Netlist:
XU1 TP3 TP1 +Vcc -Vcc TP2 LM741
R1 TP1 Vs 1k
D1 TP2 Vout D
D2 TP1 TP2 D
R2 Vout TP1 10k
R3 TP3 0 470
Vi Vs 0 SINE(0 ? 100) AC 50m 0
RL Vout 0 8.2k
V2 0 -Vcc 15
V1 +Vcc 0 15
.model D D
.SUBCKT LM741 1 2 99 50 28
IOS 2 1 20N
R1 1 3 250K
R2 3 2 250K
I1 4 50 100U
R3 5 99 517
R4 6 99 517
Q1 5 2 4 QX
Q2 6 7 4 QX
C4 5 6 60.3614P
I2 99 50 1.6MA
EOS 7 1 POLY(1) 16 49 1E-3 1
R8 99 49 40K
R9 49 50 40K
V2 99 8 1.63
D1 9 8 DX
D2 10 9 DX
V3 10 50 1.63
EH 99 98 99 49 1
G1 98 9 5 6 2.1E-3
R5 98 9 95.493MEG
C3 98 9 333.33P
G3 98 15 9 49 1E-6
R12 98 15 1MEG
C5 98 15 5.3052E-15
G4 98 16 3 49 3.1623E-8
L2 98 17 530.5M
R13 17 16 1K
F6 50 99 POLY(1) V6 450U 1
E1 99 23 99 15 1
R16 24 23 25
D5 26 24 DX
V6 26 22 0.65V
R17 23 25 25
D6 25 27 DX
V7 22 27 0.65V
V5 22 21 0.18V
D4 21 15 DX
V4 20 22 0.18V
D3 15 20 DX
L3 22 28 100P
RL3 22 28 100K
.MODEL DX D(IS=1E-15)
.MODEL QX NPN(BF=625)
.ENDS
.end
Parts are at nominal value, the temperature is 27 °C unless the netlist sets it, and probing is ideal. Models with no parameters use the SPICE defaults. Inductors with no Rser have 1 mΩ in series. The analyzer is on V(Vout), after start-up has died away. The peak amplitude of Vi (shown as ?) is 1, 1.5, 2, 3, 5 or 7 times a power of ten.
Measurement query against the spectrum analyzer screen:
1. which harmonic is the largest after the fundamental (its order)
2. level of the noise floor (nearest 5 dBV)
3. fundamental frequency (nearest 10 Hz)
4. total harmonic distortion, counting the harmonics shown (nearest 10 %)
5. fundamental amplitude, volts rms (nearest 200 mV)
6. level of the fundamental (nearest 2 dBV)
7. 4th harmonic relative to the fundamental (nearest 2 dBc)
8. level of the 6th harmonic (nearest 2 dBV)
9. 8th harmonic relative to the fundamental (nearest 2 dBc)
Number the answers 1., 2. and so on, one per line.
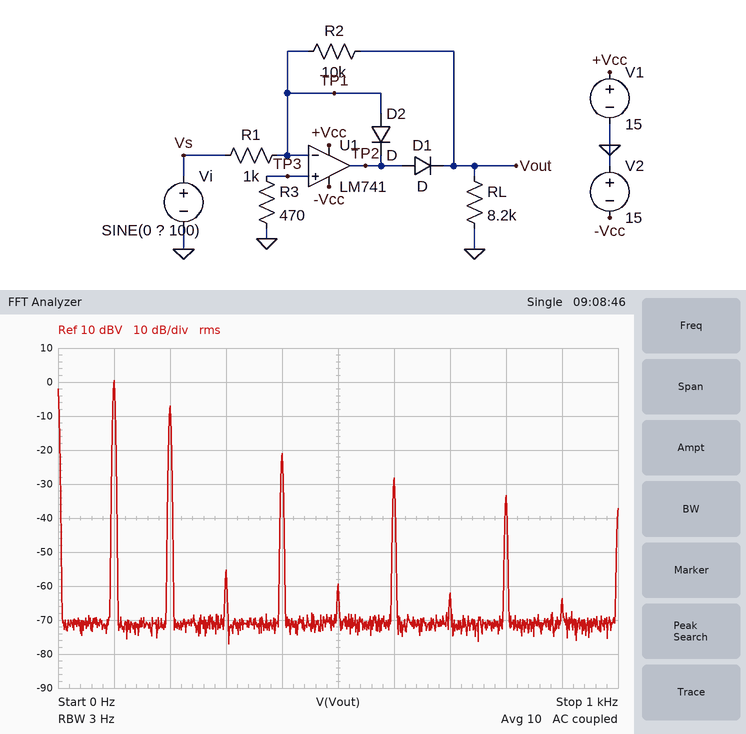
1. 2
2. -70 dBV
3. 100 Hz
4. 40 %
5. 1.0 V
6. 0 dBV
7. -22 dBc
8. -28 dBV
9. -34 dBc
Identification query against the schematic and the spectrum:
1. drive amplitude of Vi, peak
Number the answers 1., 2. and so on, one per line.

1. 300 mV
